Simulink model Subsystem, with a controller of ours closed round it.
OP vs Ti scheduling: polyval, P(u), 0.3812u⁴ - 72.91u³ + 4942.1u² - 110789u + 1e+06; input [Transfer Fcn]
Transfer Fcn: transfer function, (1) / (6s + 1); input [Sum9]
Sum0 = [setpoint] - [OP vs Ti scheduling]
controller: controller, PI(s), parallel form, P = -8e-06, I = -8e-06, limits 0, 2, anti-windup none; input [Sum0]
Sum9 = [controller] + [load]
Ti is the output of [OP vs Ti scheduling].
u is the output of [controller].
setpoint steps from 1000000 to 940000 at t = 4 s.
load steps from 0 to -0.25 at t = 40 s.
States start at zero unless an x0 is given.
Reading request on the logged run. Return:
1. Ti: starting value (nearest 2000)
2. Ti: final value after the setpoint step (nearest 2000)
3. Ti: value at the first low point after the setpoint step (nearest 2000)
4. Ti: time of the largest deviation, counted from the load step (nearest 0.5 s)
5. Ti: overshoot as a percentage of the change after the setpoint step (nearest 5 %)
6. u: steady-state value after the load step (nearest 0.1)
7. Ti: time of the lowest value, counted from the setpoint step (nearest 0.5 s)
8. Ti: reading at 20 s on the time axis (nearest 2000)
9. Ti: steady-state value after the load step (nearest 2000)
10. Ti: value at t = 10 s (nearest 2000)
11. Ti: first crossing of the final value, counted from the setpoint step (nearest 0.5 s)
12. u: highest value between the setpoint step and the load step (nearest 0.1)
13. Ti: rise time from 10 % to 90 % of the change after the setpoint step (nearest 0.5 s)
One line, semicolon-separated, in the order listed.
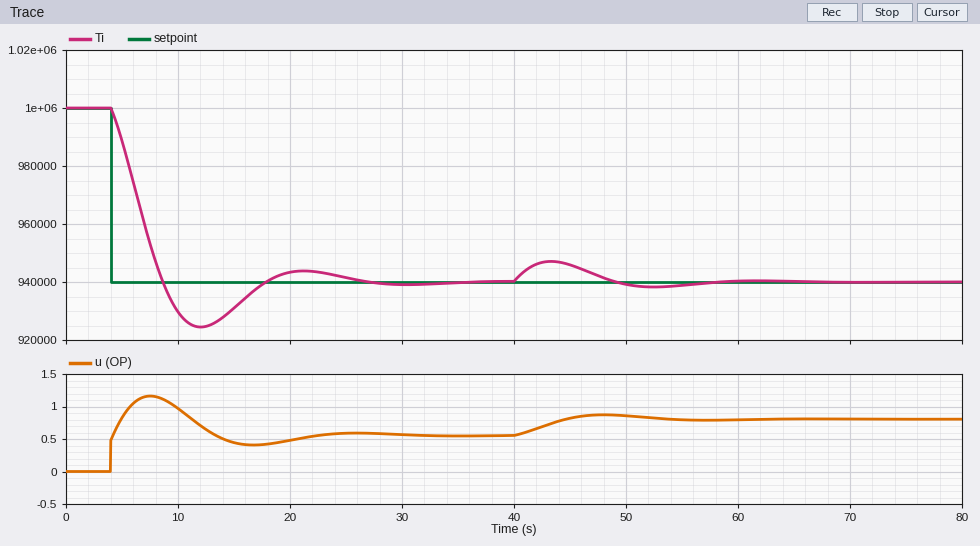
1000000; 940000; 924000; 3.5 s; 25 %; 0.8; 8.0 s; 944000; 940000; 930000; 4.5 s; 1.2; 3.5 s
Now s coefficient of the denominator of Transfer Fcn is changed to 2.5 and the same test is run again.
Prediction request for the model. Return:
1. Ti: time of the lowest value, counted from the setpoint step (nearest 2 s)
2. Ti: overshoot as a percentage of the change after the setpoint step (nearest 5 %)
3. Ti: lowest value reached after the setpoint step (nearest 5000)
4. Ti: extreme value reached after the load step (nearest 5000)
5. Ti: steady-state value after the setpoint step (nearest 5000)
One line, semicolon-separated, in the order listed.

6 s; 10 %; 935000; 950000; 940000
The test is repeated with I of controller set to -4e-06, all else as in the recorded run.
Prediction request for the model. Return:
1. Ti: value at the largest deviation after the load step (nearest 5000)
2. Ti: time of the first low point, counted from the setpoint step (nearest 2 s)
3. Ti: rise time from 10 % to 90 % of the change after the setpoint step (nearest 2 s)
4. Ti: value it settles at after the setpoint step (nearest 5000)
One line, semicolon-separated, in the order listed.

950000; 12 s; 6 s; 940000
